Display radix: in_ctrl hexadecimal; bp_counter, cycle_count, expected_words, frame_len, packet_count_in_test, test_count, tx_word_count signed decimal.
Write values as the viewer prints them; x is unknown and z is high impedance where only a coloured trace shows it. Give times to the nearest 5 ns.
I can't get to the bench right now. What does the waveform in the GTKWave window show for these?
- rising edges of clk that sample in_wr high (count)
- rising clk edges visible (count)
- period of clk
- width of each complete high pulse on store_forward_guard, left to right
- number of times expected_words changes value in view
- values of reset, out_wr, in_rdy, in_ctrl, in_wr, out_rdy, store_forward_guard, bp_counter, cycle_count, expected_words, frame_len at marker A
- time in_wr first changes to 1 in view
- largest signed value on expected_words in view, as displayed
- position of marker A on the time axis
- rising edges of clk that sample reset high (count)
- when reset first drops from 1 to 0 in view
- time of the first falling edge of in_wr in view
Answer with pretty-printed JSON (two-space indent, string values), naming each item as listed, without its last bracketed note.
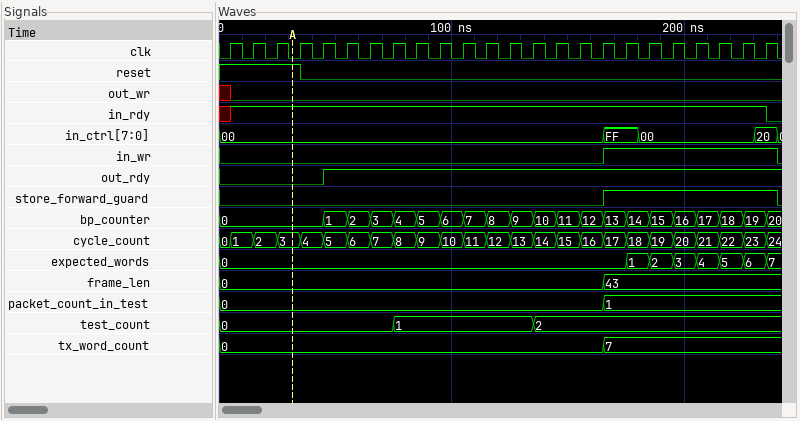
{
  "rising edges of clk that sample in_wr high": "7",
  "rising clk edges visible": "24",
  "period of clk": "10 ns",
  "width of each complete high pulse on store_forward_guard, left to right": "75 ns",
  "number of times expected_words changes value in view": "7",
  "values of reset, out_wr, in_rdy, in_ctrl, in_wr, out_rdy, store_forward_guard, bp_counter, cycle_count, expected_words, frame_len at marker A": "reset=1, out_wr=0, in_rdy=1, in_ctrl=00, in_wr=0, out_rdy=0, store_forward_guard=0, bp_counter=0, cycle_count=3, expected_words=0, frame_len=0",
  "time in_wr first changes to 1 in view": "165 ns",
  "largest signed value on expected_words in view, as displayed": "7",
  "position of marker A on the time axis": "30 ns",
  "rising edges of clk that sample reset high": "4",
  "when reset first drops from 1 to 0 in view": "35 ns",
  "time of the first falling edge of in_wr in view": "240 ns"
}
